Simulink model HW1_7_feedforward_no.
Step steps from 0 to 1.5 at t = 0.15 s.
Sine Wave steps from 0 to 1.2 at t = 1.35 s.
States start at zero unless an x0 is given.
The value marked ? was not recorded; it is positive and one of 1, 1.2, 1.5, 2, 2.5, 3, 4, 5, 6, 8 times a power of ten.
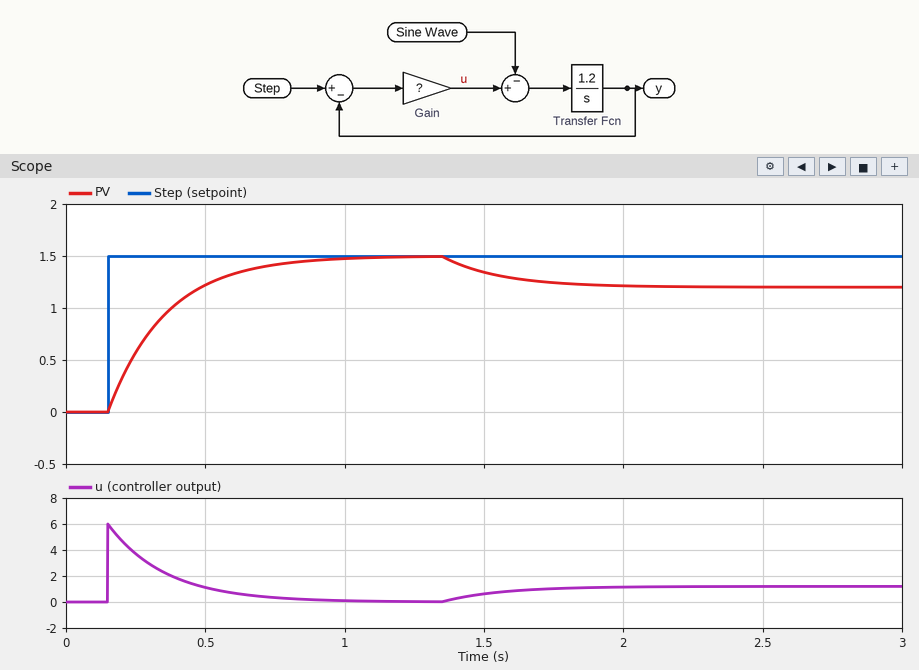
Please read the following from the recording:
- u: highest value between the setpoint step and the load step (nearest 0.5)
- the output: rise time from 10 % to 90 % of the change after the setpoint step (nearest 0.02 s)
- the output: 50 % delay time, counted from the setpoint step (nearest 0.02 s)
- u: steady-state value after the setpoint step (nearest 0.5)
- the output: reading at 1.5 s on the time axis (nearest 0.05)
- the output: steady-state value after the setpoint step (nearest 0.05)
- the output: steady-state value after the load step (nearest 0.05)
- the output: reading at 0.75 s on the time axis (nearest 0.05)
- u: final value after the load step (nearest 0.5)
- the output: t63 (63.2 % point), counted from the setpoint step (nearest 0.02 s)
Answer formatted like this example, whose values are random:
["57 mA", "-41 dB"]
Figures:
["6.0", "0.46 s", "0.14 s", "0.0", "1.35", "1.50", "1.20", "1.40", "1.0", "0.20 s"]
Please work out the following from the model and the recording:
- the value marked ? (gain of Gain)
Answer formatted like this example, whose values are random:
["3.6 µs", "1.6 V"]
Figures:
["4"]
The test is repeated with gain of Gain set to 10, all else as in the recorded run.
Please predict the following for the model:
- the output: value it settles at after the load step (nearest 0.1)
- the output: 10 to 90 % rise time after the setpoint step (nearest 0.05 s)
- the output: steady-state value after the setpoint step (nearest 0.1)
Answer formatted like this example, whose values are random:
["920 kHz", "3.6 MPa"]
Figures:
["1.4", "0.20 s", "1.5"]
